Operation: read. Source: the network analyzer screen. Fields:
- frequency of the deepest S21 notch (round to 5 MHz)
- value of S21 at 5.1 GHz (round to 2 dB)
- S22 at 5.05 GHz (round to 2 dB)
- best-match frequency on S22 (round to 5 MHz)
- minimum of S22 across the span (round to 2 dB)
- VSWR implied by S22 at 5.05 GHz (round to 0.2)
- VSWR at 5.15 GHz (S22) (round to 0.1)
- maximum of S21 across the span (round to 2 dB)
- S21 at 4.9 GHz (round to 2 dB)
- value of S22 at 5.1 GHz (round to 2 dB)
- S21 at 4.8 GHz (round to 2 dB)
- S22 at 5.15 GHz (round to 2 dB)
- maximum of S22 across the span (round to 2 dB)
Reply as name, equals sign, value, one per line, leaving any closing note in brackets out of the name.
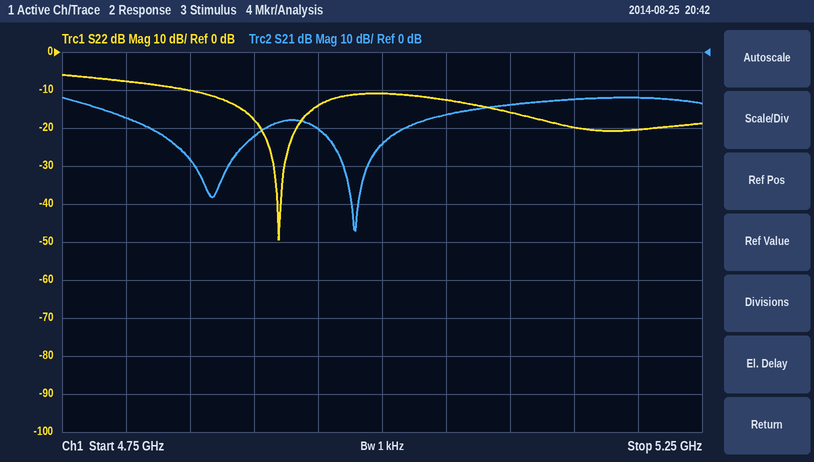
frequency of the deepest S21 notch = 4.980 GHz
value of S21 at 5.1 GHz = -14 dB
S22 at 5.05 GHz = -12 dB
best-match frequency on S22 = 4.920 GHz
minimum of S22 across the span = -50 dB
VSWR implied by S22 at 5.05 GHz = 1.6
VSWR at 5.15 GHz (S22) = 1.2
maximum of S21 across the span = -12 dB
S21 at 4.9 GHz = -22 dB
value of S22 at 5.1 GHz = -16 dB
S21 at 4.8 GHz = -18 dB
S22 at 5.15 GHz = -20 dB
maximum of S22 across the span = -6 dB
